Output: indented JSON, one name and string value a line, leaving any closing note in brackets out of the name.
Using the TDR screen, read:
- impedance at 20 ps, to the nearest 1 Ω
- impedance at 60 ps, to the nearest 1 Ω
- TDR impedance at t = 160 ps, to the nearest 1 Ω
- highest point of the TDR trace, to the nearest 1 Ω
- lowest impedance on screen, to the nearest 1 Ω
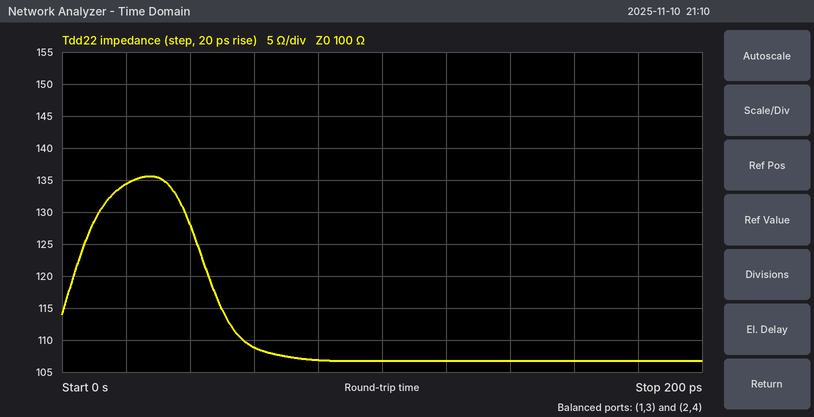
{
  "impedance at 20 ps, to the nearest 1 Ω": "134 Ω",
  "impedance at 60 ps, to the nearest 1 Ω": "109 Ω",
  "TDR impedance at t = 160 ps, to the nearest 1 Ω": "107 Ω",
  "highest point of the TDR trace, to the nearest 1 Ω": "136 Ω",
  "lowest impedance on screen, to the nearest 1 Ω": "107 Ω"
}
